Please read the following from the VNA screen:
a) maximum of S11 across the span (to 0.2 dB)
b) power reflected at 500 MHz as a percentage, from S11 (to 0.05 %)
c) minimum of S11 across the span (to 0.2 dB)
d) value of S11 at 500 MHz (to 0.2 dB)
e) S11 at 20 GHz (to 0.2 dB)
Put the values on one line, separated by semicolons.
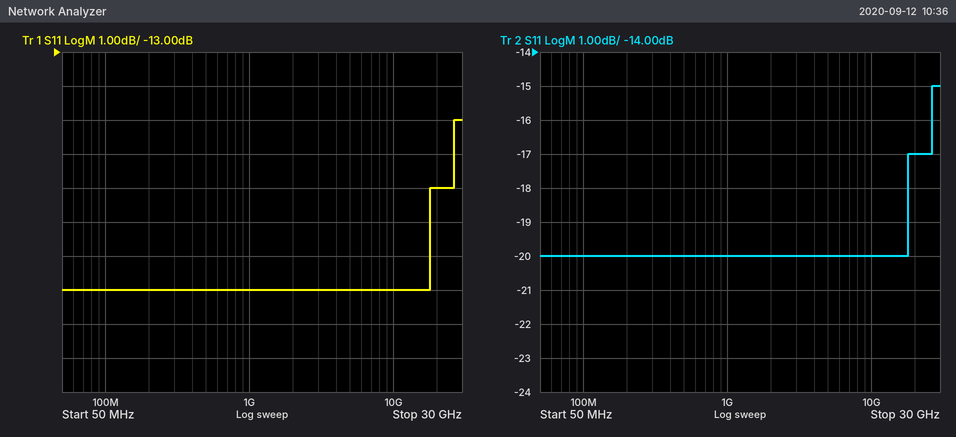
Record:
-15.0 dB; 1.00 %; -20.0 dB; -20.0 dB; -17.0 dB
